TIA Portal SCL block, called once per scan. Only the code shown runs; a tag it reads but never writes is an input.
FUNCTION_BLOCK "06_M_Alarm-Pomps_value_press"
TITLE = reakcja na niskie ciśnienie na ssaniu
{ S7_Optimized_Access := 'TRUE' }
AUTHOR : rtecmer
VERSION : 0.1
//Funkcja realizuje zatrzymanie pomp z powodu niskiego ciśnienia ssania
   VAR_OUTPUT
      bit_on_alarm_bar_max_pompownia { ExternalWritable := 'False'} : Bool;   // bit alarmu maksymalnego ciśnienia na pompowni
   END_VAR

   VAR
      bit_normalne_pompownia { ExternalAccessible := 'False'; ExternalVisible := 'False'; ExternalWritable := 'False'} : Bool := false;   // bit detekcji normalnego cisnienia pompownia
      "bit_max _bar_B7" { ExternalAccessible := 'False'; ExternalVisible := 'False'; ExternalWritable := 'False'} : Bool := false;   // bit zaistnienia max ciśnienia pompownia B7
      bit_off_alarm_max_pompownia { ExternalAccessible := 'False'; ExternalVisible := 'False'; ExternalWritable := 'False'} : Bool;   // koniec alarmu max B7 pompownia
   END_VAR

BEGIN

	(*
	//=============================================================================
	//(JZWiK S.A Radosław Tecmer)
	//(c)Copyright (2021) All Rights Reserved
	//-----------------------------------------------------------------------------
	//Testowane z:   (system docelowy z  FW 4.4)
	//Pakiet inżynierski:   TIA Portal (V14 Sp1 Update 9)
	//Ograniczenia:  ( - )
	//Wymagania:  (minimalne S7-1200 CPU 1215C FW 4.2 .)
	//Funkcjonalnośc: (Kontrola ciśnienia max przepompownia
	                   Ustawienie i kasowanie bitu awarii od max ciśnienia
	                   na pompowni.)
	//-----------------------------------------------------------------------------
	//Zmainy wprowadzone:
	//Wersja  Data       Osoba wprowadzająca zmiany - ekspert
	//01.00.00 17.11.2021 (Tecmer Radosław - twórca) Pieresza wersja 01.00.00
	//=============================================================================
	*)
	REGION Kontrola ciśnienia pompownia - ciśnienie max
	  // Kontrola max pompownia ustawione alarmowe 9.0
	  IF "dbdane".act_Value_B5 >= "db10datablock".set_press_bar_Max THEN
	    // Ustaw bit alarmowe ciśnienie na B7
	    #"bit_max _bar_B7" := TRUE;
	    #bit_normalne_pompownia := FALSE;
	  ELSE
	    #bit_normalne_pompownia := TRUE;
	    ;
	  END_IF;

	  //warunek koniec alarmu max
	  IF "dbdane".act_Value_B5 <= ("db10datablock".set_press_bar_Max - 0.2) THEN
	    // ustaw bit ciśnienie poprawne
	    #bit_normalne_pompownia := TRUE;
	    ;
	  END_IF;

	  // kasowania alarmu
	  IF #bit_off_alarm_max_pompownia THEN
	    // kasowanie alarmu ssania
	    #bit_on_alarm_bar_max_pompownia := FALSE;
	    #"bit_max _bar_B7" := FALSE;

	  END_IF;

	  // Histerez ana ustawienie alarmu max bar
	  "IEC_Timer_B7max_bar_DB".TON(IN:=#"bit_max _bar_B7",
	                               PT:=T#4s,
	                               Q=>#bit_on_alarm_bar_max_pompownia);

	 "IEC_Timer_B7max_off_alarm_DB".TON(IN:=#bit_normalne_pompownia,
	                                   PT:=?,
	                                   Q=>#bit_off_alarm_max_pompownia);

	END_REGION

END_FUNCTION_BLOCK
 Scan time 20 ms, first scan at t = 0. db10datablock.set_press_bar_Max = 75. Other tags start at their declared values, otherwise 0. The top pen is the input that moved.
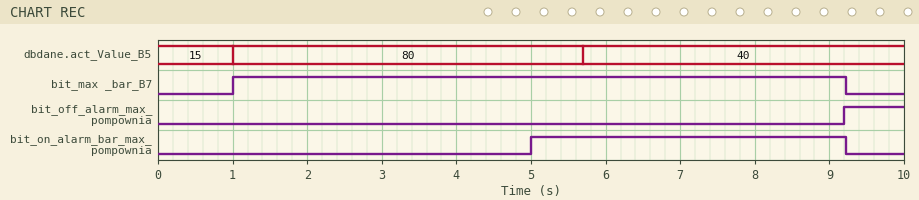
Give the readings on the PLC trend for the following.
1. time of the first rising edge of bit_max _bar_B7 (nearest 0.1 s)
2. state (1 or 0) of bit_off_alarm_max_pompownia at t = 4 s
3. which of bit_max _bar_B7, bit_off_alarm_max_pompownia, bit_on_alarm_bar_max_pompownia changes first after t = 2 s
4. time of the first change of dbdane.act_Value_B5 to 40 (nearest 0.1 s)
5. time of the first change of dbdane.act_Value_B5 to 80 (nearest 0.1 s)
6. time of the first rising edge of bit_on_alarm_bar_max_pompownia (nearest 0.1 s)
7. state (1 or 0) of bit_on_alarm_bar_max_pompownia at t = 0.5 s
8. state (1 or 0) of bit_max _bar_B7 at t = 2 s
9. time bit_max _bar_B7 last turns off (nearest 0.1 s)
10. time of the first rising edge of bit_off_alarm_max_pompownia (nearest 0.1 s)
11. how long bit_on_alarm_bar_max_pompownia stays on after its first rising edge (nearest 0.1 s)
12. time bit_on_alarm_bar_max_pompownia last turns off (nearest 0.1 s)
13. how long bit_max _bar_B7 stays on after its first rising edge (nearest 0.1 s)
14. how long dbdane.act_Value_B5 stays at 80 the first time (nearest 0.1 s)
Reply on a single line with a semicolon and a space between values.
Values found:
1.0 s; 0; bit_on_alarm_bar_max_pompownia; 5.7 s; 1.0 s; 5.0 s; 0; 1; 9.2 s; 9.2 s; 4.2 s; 9.2 s; 8.2 s; 4.7 s
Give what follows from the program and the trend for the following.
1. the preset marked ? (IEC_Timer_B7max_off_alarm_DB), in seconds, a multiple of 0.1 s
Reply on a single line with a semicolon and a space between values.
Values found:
3.5 s
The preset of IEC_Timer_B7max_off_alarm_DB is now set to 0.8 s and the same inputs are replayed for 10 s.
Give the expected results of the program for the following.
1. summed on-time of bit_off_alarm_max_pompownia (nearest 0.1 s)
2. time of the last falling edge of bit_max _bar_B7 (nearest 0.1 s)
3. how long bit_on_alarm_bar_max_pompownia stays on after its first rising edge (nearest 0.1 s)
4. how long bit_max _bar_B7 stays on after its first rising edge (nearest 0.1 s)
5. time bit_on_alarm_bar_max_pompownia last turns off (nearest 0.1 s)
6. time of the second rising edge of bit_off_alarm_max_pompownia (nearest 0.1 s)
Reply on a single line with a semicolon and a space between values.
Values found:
3.7 s; 6.5 s; 1.5 s; 5.5 s; 6.5 s; 6.5 s
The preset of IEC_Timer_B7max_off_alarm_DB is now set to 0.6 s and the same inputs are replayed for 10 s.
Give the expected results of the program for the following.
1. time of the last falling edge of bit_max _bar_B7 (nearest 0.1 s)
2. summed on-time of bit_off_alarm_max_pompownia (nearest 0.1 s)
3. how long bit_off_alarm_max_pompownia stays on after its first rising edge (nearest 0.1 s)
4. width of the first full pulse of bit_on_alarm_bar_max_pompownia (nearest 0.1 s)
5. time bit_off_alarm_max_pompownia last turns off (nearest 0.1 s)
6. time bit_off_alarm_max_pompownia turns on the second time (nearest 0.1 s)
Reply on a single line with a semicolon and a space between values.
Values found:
6.3 s; 4.1 s; 0.4 s; 1.3 s; 1.0 s; 6.3 s
